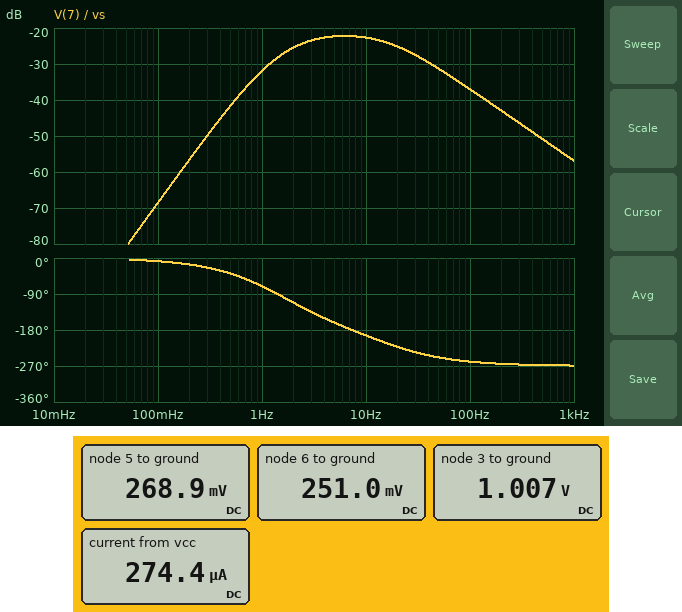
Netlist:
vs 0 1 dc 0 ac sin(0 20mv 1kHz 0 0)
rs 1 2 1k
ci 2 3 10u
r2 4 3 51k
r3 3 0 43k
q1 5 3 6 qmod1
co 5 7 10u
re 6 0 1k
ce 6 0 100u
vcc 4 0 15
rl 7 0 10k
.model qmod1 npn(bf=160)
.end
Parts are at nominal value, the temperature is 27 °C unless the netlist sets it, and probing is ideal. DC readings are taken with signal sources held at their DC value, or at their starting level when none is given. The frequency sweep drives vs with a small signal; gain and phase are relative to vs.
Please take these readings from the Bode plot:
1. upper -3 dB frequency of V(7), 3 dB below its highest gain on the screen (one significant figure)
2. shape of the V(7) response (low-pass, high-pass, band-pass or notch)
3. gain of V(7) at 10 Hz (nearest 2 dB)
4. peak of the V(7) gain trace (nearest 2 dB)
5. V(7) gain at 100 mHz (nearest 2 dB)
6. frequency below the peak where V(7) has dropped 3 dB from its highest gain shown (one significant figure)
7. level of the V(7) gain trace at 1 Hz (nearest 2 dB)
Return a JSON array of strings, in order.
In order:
["20 Hz", "band-pass", "-22 dB", "-22 dB", "-68 dB", "2 Hz", "-32 dB"]
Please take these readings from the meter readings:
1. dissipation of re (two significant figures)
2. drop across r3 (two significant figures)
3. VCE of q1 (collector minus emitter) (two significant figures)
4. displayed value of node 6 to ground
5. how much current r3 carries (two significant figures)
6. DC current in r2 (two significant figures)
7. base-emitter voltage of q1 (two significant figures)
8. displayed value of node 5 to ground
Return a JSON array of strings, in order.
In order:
["63 µW", "1.0 V", "18 mV", "251.0 mV", "23 µA", "270 µA", "760 mV", "268.9 mV"]
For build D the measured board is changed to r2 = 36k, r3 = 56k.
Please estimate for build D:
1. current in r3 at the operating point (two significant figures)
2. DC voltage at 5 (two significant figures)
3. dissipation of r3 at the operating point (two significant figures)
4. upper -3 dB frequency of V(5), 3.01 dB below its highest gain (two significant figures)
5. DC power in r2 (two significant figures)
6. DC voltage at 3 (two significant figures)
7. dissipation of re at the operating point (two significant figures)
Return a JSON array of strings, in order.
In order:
["20 µA", "380 mV", "23 µW", "20 Hz", "5.3 mW", "1.1 V", "130 µW"]
